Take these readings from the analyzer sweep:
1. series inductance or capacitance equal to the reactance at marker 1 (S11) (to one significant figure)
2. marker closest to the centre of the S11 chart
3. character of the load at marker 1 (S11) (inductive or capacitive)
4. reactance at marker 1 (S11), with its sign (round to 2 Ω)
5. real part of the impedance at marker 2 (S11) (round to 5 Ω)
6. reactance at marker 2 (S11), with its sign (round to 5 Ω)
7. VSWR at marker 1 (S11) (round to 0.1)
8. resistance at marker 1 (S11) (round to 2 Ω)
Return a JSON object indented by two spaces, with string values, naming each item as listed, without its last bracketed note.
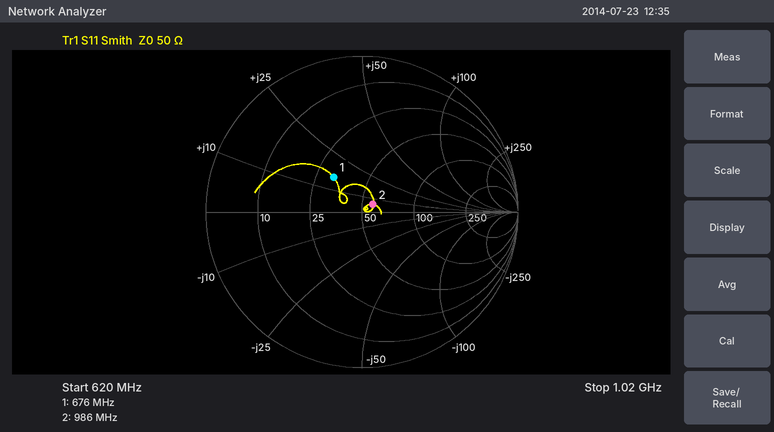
{
  "series inductance or capacitance equal to the reactance at marker 1 (S11)": "4 nH",
  "marker closest to the centre of the S11 chart": "marker 2",
  "character of the load at marker 1 (S11)": "inductive",
  "reactance at marker 1 (S11), with its sign": "+16 Ω",
  "real part of the impedance at marker 2 (S11)": "55 Ω",
  "reactance at marker 2 (S11), with its sign": "+5 Ω",
  "VSWR at marker 1 (S11)": "1.8",
  "resistance at marker 1 (S11)": "32 Ω"
}
